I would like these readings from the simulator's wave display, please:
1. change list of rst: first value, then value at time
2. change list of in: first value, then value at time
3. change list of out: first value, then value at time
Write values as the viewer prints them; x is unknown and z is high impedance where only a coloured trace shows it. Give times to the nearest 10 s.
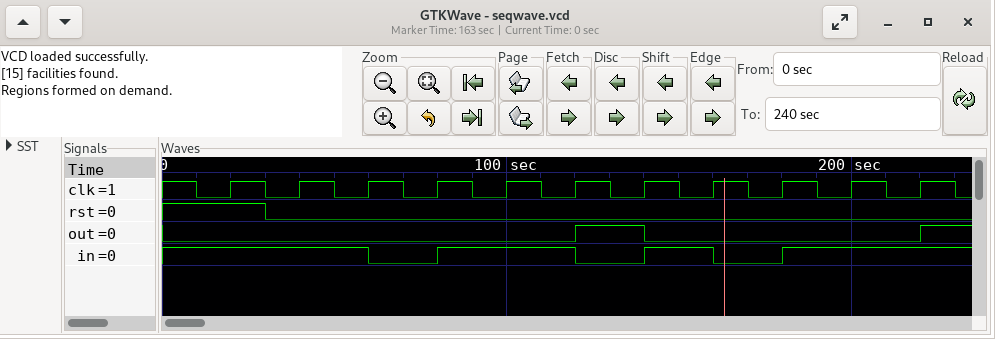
1, 0 at 30 s
1, 0 at 60 s, 1 at 80 s, 0 at 120 s, 1 at 140 s, 0 at 160 s, 1 at 180 s
0, 1 at 120 s, 0 at 140 s, 1 at 220 s
